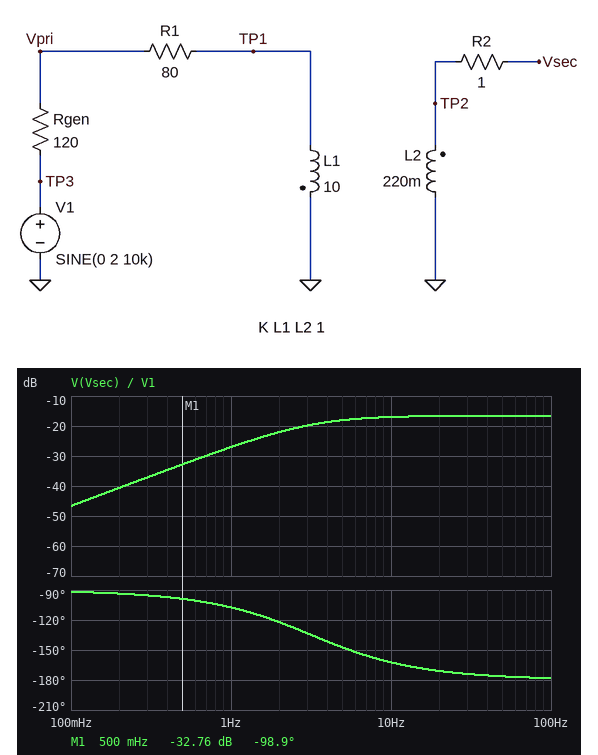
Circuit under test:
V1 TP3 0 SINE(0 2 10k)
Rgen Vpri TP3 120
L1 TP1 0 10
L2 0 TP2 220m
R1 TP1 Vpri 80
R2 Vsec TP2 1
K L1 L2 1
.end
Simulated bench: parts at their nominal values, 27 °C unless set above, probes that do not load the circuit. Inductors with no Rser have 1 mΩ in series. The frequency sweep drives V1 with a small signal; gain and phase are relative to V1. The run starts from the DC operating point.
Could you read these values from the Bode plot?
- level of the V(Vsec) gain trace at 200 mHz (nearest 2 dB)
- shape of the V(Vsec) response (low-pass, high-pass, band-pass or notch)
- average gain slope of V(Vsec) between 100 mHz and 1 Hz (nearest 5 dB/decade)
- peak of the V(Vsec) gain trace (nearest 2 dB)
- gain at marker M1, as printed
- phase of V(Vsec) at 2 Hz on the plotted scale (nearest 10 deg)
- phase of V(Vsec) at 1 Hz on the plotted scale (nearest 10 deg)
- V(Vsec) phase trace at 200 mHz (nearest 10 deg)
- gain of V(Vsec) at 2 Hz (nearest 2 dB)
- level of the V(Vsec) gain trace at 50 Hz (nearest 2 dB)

-40 dB
high-pass
20 dB/decade
-16 dB
-32.76 dB
-120 deg
-110 deg
-90 deg
-22 dB
-16 dB
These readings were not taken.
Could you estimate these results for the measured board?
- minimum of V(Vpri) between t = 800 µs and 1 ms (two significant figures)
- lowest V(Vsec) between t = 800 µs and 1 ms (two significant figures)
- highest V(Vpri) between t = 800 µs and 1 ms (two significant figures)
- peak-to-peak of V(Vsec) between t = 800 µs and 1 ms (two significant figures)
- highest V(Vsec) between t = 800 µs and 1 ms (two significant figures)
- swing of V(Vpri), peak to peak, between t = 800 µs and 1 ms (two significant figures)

-2.0 V
-300 mV
2.0 V
590 mV
300 mV
4.0 V
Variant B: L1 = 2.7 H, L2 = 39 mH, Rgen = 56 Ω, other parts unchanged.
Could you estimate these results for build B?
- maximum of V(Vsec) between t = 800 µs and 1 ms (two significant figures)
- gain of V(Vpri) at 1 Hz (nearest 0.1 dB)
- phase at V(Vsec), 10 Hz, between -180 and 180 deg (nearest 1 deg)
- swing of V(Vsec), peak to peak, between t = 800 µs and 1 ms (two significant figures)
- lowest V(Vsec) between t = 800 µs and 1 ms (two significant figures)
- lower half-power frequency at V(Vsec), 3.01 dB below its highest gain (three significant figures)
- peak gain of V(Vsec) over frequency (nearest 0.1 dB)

240 mV
-4.5 dB
-141 deg
480 mV
-240 mV
8.02 Hz
-18.4 dB
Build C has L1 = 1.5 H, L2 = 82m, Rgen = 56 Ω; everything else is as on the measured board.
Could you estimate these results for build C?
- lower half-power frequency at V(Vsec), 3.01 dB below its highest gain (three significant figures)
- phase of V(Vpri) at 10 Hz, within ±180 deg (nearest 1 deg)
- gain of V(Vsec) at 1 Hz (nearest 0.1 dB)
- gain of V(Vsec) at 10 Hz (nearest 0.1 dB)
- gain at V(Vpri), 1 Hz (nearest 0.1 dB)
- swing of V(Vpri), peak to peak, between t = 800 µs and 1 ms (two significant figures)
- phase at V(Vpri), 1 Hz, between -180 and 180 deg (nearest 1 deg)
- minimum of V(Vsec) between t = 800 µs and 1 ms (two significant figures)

14.4 Hz
15 deg
-35.8 dB
-17.5 dB
-4.6 dB
4.0 V
3 deg
-470 mV
